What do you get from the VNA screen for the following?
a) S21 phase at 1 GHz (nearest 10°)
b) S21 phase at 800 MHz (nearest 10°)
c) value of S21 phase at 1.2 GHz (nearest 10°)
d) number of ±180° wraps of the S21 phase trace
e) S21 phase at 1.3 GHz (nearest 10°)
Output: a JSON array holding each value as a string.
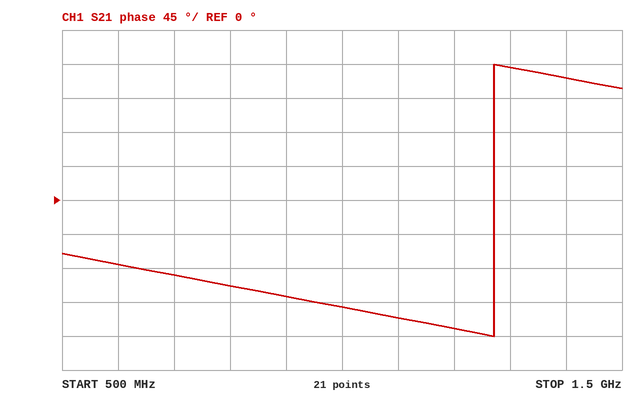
["-140°", "-110°", "-170°", "1", "180°"]
